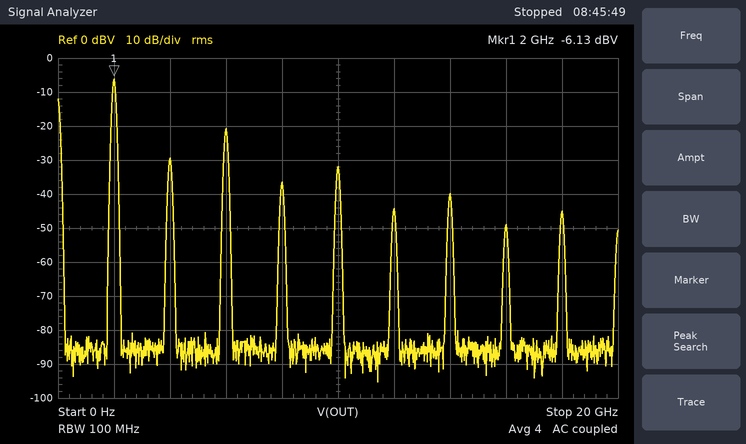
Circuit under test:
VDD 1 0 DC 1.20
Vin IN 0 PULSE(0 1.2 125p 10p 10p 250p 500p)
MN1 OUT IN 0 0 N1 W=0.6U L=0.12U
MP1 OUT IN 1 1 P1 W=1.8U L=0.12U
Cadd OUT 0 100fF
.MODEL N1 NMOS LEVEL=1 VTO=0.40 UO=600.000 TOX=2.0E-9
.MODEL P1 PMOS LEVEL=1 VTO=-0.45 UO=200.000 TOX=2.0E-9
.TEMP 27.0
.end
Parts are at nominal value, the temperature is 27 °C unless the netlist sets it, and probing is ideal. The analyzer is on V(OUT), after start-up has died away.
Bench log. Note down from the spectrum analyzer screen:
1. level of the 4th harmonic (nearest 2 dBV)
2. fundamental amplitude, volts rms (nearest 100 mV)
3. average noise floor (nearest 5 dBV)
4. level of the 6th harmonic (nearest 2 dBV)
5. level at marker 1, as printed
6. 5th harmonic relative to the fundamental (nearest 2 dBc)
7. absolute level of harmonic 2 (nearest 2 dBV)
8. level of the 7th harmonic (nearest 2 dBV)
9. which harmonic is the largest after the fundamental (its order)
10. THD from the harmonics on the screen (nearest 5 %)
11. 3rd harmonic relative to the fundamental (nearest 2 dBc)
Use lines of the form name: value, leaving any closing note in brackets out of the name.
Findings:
level of the 4th harmonic: -36 dBV
fundamental amplitude, volts rms: 500 mV
average noise floor: -85 dBV
level of the 6th harmonic: -44 dBV
level at marker 1, as printed: -6.13 dBV
5th harmonic relative to the fundamental: -26 dBc
absolute level of harmonic 2: -30 dBV
level of the 7th harmonic: -40 dBV
which harmonic is the largest after the fundamental: 3
THD from the harmonics on the screen: 20 %
3rd harmonic relative to the fundamental: -14 dBc
